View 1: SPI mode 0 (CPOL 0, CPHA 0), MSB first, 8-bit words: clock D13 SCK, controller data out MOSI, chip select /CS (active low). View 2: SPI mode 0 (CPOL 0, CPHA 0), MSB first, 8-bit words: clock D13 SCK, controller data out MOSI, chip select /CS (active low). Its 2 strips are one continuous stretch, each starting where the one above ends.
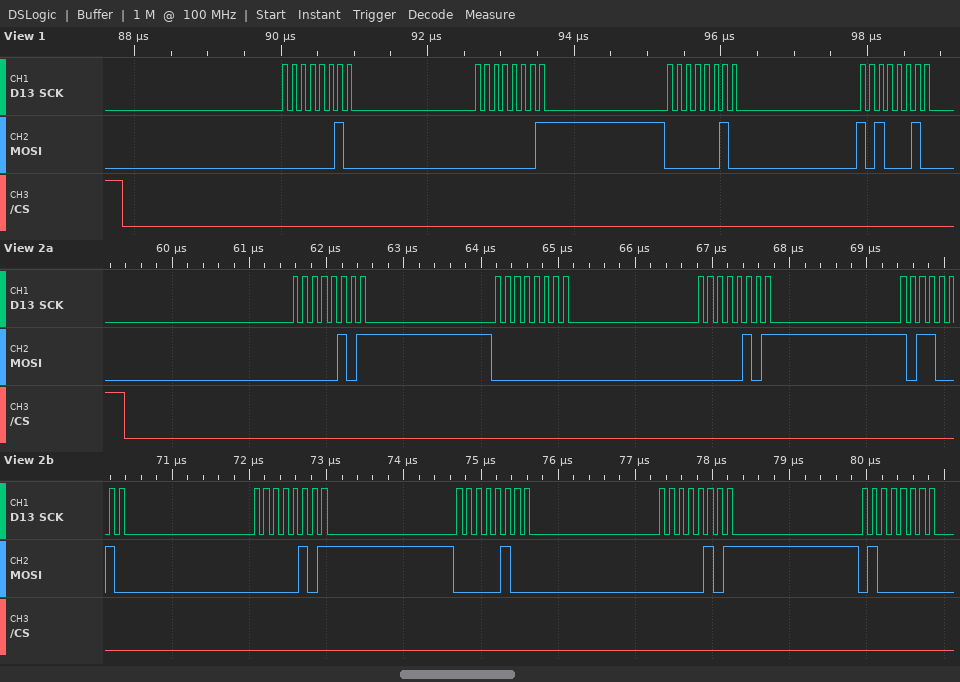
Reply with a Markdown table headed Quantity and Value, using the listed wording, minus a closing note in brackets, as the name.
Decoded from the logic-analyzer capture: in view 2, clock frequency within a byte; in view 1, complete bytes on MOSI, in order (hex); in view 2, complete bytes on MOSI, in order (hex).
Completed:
| Quantity | Value |
|---|---|
| in view 2, clock frequency within a byte | 8 MHz |
| in view 1, complete bytes on MOSI, in order | 02 01 02 A2 |
| in view 2, complete bytes on MOSI, in order | 0x05 0x00 0x05 0xB2 0x05 0x04 0x05 0x40 |
